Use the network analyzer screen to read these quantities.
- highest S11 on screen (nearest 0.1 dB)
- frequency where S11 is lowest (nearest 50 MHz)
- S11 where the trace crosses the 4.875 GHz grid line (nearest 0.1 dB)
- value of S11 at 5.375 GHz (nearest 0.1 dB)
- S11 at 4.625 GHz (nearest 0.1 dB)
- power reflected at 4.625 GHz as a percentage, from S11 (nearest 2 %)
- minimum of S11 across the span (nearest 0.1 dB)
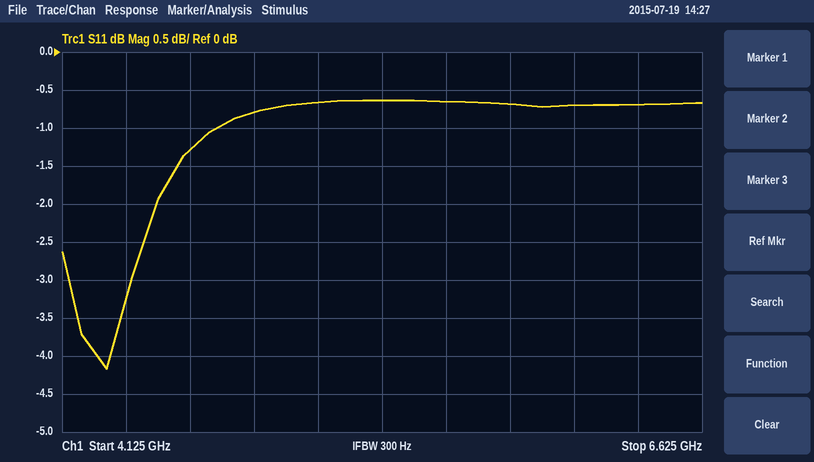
-0.6 dB
4.30 GHz
-0.8 dB
-0.6 dB
-1.3 dB
74 %
-4.2 dB
